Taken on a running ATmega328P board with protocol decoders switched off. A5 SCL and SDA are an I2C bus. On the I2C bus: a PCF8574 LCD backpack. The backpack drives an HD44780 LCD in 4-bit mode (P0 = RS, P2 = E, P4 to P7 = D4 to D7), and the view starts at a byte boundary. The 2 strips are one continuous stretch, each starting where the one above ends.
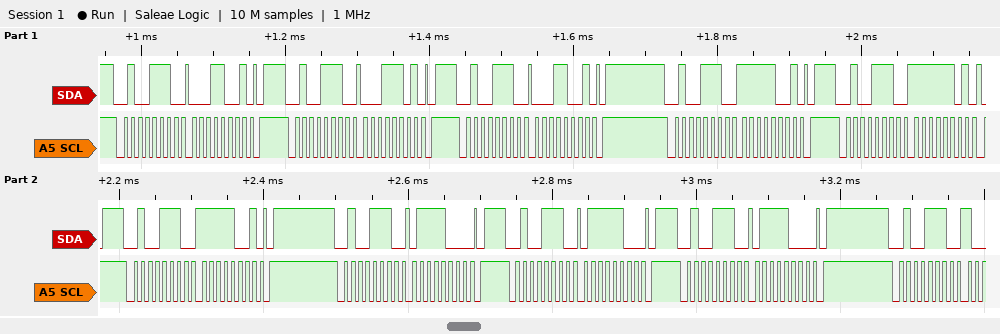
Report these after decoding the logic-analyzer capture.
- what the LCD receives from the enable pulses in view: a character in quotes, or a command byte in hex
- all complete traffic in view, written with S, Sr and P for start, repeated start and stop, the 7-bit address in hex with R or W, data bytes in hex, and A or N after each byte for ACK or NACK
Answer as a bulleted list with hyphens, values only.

- data 0x1F
- S 27W A 19 A P S 27W A 1D A P S 27W A 19 A P S 27W A F9 A P S 27W A FD A P S 27W A F9 A P S 27W A 78 A P S 27W A 7C A P S 27W A 78 A P S 27W A
